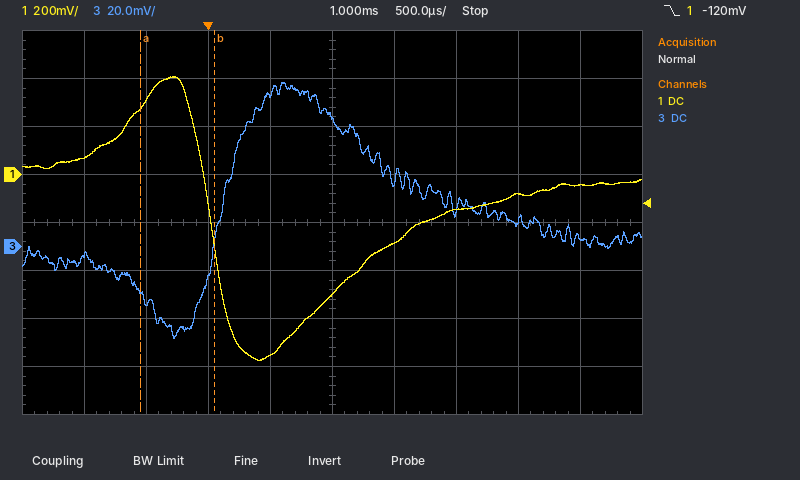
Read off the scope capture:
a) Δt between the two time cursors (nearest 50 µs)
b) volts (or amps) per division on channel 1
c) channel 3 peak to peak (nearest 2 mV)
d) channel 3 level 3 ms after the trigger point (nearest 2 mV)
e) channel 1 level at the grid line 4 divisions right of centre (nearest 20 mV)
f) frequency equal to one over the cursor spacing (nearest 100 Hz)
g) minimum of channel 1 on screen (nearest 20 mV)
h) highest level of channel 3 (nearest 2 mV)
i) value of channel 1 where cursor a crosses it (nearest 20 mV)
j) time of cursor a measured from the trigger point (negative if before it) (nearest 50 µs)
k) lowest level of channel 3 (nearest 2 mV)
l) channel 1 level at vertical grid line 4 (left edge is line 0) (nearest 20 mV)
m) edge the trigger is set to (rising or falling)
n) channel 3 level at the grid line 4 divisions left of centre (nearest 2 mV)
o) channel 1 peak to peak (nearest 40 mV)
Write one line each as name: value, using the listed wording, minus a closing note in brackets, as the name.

Δt between the two time cursors: 600 µs
volts (or amps) per division on channel 1: 200 mV
channel 3 peak to peak: 106 mV
channel 3 level 3 ms after the trigger point: 4 mV
channel 1 level at the grid line 4 divisions right of centre: -40 mV
frequency equal to one over the cursor spacing: 1.7 kHz
minimum of channel 1 on screen: -780 mV
highest level of channel 3: 68 mV
value of channel 1 where cursor a crosses it: 280 mV
time of cursor a measured from the trigger point (negative if before it): -550 µs
lowest level of channel 3: -38 mV
channel 1 level at vertical grid line 4 (left edge is line 0): -760 mV
edge the trigger is set to: falling
channel 3 level at the grid line 4 divisions left of centre: -4 mV
channel 1 peak to peak: 1.20 V
